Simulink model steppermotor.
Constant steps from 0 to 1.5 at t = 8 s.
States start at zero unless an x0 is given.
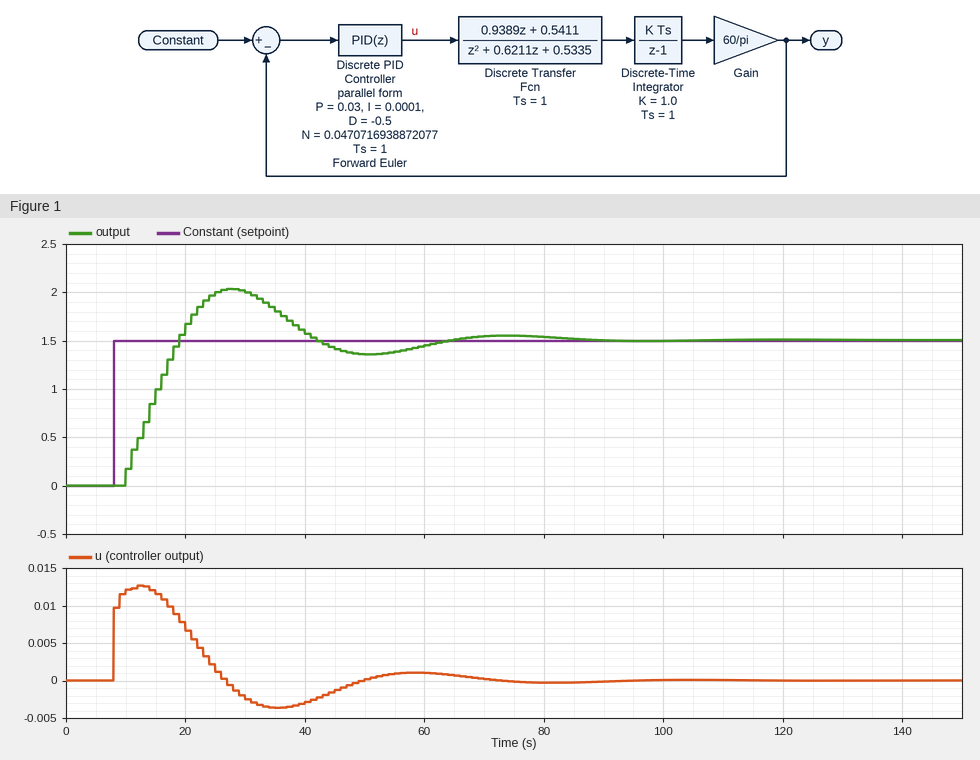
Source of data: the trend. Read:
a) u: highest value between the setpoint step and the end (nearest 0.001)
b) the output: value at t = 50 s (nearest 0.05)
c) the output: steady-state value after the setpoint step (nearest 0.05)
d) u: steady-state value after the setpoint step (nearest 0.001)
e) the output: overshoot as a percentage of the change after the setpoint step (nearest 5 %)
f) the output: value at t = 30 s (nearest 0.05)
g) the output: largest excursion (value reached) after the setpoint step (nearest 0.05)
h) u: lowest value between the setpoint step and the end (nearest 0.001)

0.013
1.35
1.50
0.000
35 %
2.00
2.05
-0.004
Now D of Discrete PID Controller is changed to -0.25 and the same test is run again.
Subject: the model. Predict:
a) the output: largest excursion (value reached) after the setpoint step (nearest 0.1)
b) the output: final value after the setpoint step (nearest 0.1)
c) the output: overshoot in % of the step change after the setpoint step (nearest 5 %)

1.6
1.5
10 %
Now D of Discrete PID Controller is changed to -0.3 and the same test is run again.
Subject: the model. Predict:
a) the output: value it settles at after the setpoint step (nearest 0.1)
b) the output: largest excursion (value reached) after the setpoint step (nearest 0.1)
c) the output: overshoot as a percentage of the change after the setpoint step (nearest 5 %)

1.5
1.7
10 %
